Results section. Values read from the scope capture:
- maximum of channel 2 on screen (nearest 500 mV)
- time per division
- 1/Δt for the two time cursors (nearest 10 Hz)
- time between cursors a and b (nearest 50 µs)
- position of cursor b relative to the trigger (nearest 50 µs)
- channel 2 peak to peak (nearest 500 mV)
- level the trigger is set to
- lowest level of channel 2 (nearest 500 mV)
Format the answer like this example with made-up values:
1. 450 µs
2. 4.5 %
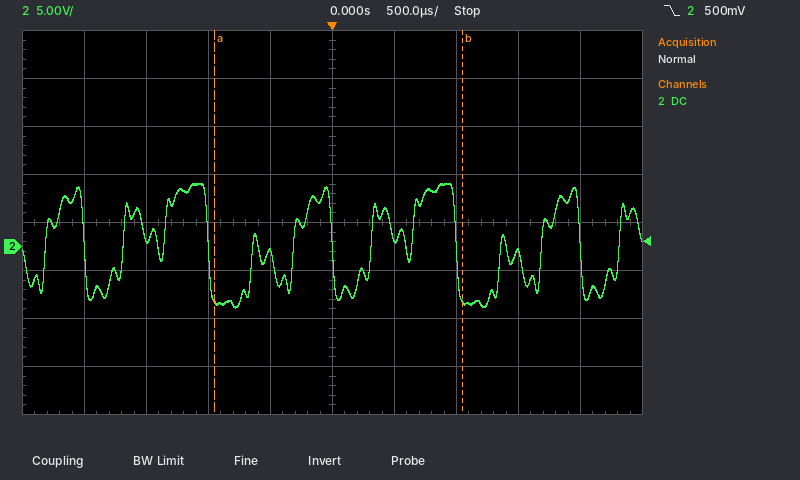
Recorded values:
1. 6.5 V
2. 500 µs
3. 500 Hz
4. 2.00 ms
5. +1.05 ms
6. 13.0 V
7. 500 mV
8. -6.5 V
